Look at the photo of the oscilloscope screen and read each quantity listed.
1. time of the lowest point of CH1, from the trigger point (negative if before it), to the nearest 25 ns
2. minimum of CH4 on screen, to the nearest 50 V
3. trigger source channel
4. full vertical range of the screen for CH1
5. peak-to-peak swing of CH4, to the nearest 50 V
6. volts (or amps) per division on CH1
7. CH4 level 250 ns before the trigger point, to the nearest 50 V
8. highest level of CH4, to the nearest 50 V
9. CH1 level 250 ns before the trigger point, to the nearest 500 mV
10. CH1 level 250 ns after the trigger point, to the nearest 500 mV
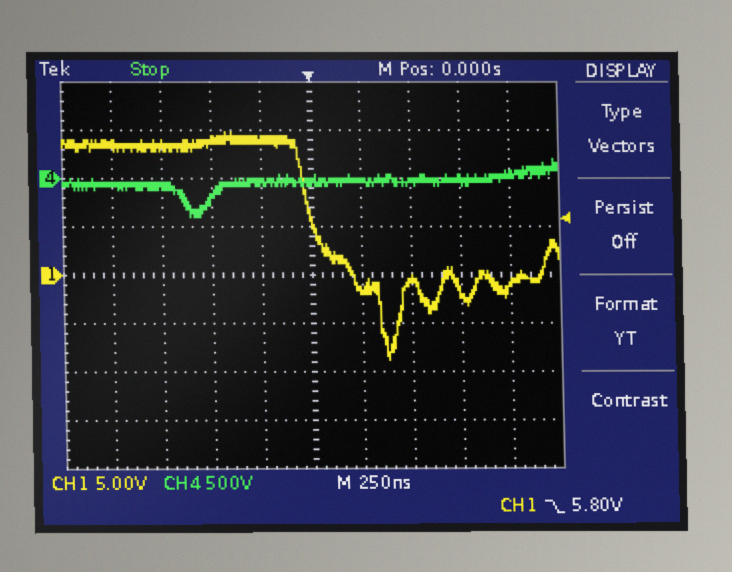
+375 ns
-400 V
CH1
40 V
600 V
5 V
-50 V
200 V
14.0 V
-1.5 V
